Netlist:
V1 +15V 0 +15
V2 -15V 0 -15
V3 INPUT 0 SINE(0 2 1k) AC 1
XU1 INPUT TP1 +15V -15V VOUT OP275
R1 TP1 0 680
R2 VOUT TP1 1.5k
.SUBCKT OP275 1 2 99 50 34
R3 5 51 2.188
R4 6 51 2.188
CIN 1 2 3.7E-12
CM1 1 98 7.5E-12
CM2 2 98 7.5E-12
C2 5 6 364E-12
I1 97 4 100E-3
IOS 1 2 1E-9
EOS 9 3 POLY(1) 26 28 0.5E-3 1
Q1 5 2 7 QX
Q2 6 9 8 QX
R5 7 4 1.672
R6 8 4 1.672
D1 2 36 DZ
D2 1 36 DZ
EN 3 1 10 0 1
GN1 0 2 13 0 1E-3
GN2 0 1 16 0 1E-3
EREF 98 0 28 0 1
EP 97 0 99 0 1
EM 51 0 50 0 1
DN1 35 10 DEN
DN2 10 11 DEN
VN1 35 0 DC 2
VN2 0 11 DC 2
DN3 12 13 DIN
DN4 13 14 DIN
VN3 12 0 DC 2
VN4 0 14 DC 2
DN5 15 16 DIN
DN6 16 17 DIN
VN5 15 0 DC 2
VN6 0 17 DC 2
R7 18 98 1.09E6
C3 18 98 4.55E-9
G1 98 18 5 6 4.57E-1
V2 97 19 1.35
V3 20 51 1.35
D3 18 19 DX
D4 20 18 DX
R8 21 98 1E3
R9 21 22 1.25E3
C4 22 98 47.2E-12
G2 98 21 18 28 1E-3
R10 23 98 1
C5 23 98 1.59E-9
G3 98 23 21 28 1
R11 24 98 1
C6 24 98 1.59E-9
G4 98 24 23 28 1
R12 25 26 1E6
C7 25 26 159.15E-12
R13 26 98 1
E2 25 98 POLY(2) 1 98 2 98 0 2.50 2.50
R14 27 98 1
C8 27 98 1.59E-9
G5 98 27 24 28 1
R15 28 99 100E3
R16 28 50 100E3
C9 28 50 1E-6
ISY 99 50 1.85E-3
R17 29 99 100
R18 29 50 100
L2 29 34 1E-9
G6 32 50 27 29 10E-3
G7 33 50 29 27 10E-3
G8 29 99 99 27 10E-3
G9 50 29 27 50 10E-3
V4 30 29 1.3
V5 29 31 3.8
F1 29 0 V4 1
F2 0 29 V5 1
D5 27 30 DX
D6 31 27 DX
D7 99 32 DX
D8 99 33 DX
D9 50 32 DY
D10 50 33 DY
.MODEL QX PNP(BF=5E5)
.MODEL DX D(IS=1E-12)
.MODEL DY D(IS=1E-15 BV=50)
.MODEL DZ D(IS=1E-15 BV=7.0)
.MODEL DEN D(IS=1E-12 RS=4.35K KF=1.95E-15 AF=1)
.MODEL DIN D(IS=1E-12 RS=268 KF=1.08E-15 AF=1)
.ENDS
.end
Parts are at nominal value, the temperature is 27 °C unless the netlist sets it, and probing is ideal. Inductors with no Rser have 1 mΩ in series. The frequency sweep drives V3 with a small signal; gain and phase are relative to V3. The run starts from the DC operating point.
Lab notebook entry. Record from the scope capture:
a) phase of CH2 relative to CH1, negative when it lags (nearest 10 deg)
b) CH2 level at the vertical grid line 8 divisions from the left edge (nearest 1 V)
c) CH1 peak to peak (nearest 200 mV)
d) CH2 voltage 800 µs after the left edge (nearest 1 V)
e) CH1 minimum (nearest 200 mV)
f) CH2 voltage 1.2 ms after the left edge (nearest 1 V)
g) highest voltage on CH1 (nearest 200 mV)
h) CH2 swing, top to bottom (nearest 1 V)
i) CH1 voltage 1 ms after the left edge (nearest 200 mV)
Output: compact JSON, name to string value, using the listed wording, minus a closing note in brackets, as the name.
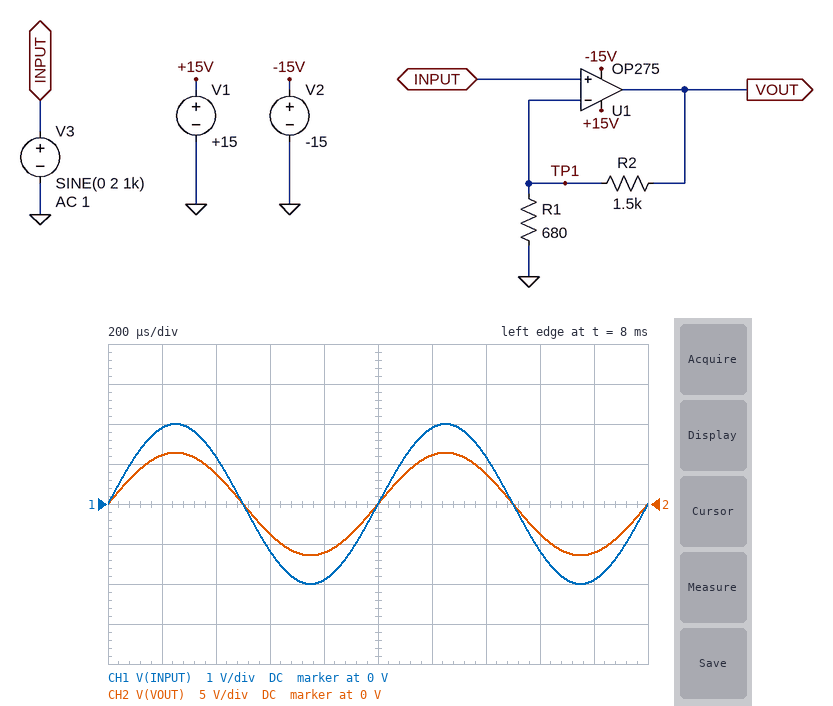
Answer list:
{"phase of CH2 relative to CH1, negative when it lags": "0 deg", "CH2 level at the vertical grid line 8 divisions from the left edge": "-4 V", "CH1 peak to peak": "4.0 V", "CH2 voltage 800 µs after the left edge": "-6 V", "CH1 minimum": "-2.0 V", "CH2 voltage 1.2 ms after the left edge": "6 V", "highest voltage on CH1": "2.0 V", "CH2 swing, top to bottom": "13 V", "CH1 voltage 1 ms after the left edge": "0 V"}
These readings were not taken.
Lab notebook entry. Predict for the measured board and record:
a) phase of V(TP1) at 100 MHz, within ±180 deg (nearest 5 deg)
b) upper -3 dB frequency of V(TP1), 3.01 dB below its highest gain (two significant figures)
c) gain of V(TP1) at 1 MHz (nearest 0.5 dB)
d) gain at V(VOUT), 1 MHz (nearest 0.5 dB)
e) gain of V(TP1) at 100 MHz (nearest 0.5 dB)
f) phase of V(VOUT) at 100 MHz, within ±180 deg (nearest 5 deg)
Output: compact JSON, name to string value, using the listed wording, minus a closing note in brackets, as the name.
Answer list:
{"phase of V(TP1) at 100 MHz, within ±180 deg": "15 deg", "upper -3 dB frequency of V(TP1), 3.01 dB below its highest gain": "4.2 MHz", "gain of V(TP1) at 1 MHz": "0.5 dB", "gain at V(VOUT), 1 MHz": "10.5 dB", "gain of V(TP1) at 100 MHz": "-10.0 dB", "phase of V(VOUT) at 100 MHz, within ±180 deg": "75 deg"}
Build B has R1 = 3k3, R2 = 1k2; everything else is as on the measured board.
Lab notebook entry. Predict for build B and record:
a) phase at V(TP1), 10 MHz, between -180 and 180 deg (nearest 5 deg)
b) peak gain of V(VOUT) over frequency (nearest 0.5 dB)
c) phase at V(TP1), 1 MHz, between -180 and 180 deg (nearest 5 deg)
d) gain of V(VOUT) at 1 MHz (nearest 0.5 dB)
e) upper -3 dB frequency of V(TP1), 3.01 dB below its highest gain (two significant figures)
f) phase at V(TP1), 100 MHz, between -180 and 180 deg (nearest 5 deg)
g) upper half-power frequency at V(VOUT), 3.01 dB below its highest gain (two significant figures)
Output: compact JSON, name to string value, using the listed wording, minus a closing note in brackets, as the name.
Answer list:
{"phase at V(TP1), 10 MHz, between -180 and 180 deg": "-135 deg", "peak gain of V(VOUT) over frequency": "5.5 dB", "phase at V(TP1), 1 MHz, between -180 and 180 deg": "-5 deg", "gain of V(VOUT) at 1 MHz": "3.0 dB", "upper -3 dB frequency of V(TP1), 3.01 dB below its highest gain": "8.9 MHz", "phase at V(TP1), 100 MHz, between -180 and 180 deg": "10 deg", "upper half-power frequency at V(VOUT), 3.01 dB below its highest gain": "10 MHz"}
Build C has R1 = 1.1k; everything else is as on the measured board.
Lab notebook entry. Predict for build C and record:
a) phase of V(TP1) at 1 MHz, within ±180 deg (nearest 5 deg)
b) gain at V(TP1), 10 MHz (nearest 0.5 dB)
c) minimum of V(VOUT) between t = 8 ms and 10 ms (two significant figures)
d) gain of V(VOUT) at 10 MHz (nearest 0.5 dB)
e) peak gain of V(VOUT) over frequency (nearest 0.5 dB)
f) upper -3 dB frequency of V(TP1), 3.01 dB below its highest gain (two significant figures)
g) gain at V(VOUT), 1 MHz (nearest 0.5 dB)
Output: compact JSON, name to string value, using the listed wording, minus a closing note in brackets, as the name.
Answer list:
{"phase of V(TP1) at 1 MHz, within ±180 deg": "-10 deg", "gain at V(TP1), 10 MHz": "-10.5 dB", "minimum of V(VOUT) between t = 8 ms and 10 ms": "-4.7 V", "gain of V(VOUT) at 10 MHz": "1.0 dB", "peak gain of V(VOUT) over frequency": "8.5 dB", "upper -3 dB frequency of V(TP1), 3.01 dB below its highest gain": "5.5 MHz", "gain at V(VOUT), 1 MHz": "8.0 dB"}
